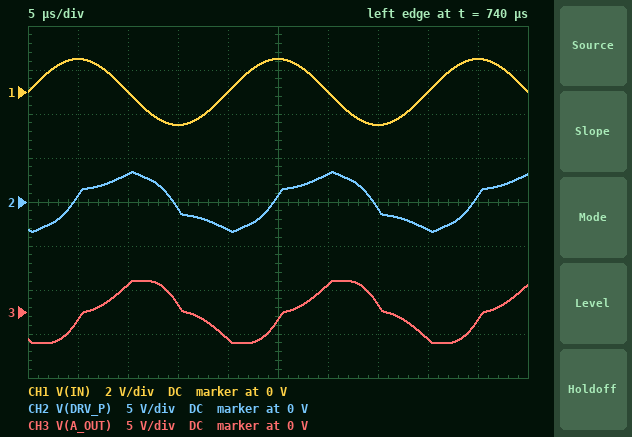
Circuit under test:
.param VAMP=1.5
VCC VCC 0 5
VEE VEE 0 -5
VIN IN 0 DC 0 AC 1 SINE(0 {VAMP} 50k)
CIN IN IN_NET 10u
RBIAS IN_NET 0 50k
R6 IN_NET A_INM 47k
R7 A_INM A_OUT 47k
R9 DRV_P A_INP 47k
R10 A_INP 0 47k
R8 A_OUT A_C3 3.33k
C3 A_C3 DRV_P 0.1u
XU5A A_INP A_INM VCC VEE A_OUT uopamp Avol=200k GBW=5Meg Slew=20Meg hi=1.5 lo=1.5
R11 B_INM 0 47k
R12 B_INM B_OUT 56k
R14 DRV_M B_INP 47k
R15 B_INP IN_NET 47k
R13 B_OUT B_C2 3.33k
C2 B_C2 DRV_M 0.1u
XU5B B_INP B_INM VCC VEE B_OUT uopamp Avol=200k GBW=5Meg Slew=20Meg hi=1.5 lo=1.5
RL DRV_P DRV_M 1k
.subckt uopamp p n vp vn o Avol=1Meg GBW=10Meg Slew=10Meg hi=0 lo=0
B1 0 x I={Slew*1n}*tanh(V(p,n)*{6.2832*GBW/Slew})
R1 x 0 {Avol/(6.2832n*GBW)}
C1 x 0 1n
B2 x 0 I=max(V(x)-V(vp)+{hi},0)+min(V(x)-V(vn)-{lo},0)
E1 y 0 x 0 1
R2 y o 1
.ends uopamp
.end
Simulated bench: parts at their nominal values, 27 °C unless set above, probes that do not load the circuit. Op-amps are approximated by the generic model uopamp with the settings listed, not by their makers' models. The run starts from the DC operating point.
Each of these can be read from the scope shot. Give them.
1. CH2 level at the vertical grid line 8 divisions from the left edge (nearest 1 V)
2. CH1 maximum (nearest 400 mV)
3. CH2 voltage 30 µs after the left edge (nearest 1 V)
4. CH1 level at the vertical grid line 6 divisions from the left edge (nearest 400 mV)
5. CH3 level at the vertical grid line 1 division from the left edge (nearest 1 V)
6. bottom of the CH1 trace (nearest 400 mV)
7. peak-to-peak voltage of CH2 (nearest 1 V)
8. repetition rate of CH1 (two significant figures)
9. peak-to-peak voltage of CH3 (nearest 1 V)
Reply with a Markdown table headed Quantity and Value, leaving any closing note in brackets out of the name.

| Quantity | Value |
|---|---|
| CH2 level at the vertical grid line 8 divisions from the left edge | -3 V |
| CH1 maximum | 1.6 V |
| CH2 voltage 30 µs after the left edge | 3 V |
| CH1 level at the vertical grid line 6 divisions from the left edge | 0 V |
| CH3 level at the vertical grid line 1 division from the left edge | -1 V |
| bottom of the CH1 trace | -1.6 V |
| peak-to-peak voltage of CH2 | 7 V |
| repetition rate of CH1 | 50 kHz |
| peak-to-peak voltage of CH3 | 7 V |
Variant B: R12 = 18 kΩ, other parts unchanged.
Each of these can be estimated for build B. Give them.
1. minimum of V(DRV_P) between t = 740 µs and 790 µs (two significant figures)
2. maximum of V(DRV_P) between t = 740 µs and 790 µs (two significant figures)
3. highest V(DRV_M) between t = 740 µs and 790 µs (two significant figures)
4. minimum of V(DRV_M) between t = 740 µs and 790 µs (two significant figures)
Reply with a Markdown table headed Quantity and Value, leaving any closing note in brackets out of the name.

| Quantity | Value |
|---|---|
| minimum of V(DRV_P) between t = 740 µs and 790 µs | -1.5 V |
| maximum of V(DRV_P) between t = 740 µs and 790 µs | 1.5 V |
| highest V(DRV_M) between t = 740 µs and 790 µs | 1.0 V |
| minimum of V(DRV_M) between t = 740 µs and 790 µs | -1.0 V |
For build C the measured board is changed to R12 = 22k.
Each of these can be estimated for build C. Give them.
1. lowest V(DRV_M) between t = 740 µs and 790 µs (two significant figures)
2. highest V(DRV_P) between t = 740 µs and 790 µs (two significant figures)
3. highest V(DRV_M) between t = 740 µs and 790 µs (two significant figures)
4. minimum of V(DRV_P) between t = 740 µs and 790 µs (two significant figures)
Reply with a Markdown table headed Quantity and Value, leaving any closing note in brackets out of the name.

| Quantity | Value |
|---|---|
| lowest V(DRV_M) between t = 740 µs and 790 µs | -970 mV |
| highest V(DRV_P) between t = 740 µs and 790 µs | 1.4 V |
| highest V(DRV_M) between t = 740 µs and 790 µs | 980 mV |
| minimum of V(DRV_P) between t = 740 µs and 790 µs | -1.4 V |
